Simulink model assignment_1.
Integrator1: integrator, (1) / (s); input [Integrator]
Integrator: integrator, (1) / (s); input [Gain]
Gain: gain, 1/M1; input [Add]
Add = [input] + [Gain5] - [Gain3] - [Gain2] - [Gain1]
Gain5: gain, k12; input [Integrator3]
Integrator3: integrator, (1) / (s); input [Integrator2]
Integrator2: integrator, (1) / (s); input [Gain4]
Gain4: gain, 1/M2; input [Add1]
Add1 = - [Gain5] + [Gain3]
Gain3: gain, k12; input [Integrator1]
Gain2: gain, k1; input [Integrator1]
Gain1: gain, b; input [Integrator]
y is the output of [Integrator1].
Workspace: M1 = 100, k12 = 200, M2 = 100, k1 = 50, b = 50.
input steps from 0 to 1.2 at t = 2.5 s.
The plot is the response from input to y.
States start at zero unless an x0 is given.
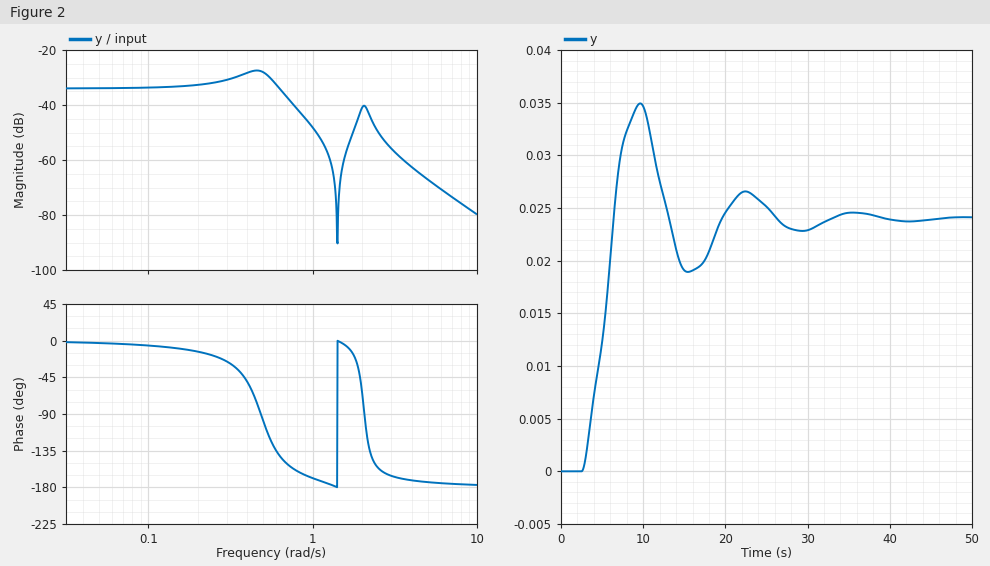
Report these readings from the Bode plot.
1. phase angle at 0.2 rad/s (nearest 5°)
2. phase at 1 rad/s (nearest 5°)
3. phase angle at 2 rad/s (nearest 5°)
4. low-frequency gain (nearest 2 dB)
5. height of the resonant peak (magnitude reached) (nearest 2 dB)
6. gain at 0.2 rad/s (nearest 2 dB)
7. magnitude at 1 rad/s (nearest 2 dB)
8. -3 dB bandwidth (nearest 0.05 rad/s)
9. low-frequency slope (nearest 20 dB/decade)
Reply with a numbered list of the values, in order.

1. -15°
2. -170°
3. -65°
4. -34 dB
5. -28 dB
6. -32 dB
7. -48 dB
8. 0.70 rad/s
9. 0 dB/decade
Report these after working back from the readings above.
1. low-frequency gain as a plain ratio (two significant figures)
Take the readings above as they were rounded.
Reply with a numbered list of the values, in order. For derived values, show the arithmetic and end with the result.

1. 10^(-34 / 20) = 0.020
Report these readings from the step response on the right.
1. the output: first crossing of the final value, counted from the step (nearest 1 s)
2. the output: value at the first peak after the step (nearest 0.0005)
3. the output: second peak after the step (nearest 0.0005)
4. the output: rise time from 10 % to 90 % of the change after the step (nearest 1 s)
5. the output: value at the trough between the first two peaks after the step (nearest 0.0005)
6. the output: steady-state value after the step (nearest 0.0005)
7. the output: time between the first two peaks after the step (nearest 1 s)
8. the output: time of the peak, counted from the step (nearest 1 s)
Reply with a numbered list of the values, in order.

1. 4 s
2. 0.0350
3. 0.0265
4. 3 s
5. 0.0190
6. 0.0240
7. 13 s
8. 7 s
